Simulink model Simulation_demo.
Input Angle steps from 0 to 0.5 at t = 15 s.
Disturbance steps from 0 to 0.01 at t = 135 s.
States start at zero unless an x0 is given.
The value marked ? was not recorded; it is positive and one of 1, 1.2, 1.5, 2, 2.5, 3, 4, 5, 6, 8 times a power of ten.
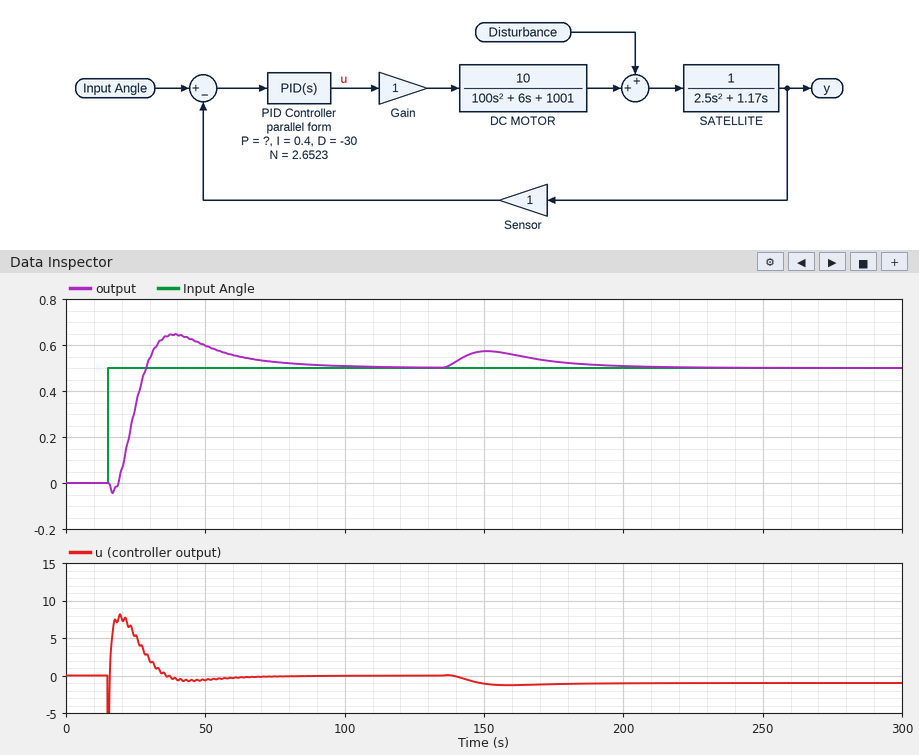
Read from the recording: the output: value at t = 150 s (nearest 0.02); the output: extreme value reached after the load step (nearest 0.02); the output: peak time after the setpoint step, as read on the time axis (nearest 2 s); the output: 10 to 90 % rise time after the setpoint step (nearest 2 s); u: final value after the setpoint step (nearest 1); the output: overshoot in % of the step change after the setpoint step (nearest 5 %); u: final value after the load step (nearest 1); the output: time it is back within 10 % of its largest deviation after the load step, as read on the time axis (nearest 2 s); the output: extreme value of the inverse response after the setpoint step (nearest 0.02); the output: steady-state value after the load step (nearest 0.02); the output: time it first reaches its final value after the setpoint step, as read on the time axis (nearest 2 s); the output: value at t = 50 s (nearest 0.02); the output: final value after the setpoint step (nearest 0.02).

0.58
0.58
40 s
8 s
0
30 %
-1
204 s
-0.04
0.50
28 s
0.60
0.50
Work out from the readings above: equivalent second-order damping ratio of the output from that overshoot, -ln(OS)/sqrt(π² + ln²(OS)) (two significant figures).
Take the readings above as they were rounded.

0.36
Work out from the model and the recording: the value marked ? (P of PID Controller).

12
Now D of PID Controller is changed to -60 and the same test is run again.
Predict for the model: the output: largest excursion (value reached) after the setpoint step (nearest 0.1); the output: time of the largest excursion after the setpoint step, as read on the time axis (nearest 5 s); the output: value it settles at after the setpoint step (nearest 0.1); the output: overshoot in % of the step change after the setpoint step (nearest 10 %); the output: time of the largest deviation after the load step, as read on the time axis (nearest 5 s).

0.8
35 s
0.5
60 %
150 s
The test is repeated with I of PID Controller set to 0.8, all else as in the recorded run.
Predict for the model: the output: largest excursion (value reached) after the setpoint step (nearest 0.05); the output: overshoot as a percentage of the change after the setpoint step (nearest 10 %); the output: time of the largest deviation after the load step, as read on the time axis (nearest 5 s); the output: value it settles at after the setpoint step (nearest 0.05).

0.75
50 %
150 s
0.50
